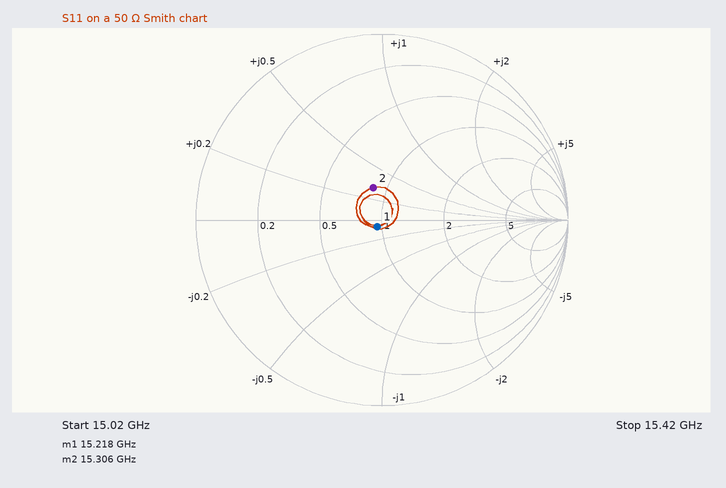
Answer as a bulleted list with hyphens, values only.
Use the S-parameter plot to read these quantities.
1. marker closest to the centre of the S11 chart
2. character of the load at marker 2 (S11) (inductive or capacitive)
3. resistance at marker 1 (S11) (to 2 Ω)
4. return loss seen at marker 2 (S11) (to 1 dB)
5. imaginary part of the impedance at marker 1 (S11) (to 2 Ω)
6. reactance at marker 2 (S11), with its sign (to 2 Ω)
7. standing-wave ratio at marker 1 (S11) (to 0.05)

- marker 1
- inductive
- 48 Ω
- 15 dB
- -4 Ω
- +16 Ω
- 1.10
